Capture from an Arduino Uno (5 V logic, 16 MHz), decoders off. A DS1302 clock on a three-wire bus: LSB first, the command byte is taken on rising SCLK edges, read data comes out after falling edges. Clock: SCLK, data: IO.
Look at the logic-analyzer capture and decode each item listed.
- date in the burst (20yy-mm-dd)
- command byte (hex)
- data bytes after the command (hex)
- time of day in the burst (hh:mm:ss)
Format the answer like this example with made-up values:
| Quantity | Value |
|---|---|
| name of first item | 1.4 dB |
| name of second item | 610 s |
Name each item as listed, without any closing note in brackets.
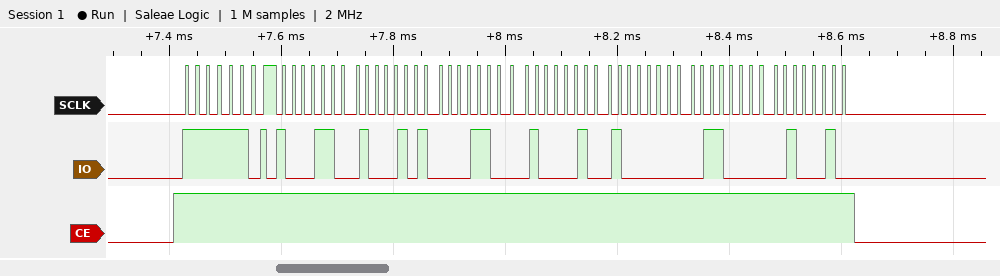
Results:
| Quantity | Value |
|---|---|
| date in the burst | 2022-01-21 |
| command byte | 0xBF |
| data bytes after the command | 31 51 18 21 01 06 22 |
| time of day in the burst | 18:51:31 |
